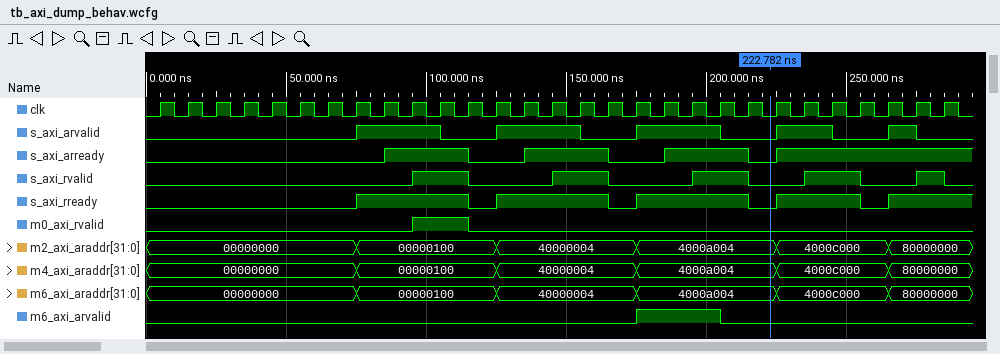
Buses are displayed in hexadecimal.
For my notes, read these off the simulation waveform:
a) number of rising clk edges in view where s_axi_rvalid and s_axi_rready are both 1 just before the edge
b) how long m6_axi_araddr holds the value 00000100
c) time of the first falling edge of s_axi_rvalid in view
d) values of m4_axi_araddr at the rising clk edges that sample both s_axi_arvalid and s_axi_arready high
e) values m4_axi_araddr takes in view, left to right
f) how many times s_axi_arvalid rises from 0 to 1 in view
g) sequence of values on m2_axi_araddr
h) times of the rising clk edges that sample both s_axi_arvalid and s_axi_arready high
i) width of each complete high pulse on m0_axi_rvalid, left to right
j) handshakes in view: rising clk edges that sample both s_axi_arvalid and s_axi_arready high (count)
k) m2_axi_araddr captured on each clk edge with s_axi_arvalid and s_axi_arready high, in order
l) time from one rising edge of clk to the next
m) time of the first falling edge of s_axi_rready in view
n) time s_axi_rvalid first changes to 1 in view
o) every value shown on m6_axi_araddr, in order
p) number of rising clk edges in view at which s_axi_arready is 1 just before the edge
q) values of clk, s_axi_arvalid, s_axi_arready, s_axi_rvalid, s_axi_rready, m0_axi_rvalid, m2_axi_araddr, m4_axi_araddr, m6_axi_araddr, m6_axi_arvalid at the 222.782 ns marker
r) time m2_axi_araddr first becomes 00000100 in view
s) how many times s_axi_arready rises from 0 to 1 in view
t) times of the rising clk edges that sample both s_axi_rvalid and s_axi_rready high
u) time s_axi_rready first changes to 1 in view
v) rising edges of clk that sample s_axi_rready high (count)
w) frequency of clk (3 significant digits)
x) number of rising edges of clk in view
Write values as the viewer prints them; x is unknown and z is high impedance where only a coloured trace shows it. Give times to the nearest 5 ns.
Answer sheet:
9
50 ns
115 ns
00000100, 00000100, 40000004, 40000004, 4000a004, 4000a004, 4000c000, 4000c000, 80000000
00000000, 00000100, 40000004, 4000a004, 4000c000, 80000000
5
00000000, 00000100, 40000004, 4000a004, 4000c000, 80000000
95 ns, 105 ns, 145 ns, 155 ns, 195 ns, 205 ns, 235 ns, 245 ns, 275 ns
20 ns
9
00000100, 00000100, 40000004, 40000004, 4000a004, 4000a004, 4000c000, 4000c000, 80000000
10 ns
115 ns
95 ns
00000000, 00000100, 40000004, 4000a004, 4000c000, 80000000
15
clk=0, s_axi_arvalid=0, s_axi_arready=0, s_axi_rvalid=0, s_axi_rready=0, m0_axi_rvalid=0, m2_axi_araddr=4000a004, m4_axi_araddr=4000a004, m6_axi_araddr=4000a004, m6_axi_arvalid=0
75 ns
4
105 ns, 115 ns, 155 ns, 165 ns, 205 ns, 215 ns, 245 ns, 255 ns, 285 ns
75 ns
17
100 MHz
29
